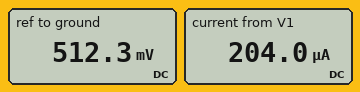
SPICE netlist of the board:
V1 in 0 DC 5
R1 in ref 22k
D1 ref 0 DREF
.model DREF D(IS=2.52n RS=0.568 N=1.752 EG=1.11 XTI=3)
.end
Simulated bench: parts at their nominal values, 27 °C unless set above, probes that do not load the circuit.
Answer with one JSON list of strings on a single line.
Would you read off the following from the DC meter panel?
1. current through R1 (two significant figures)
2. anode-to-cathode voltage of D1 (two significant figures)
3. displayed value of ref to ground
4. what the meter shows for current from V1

["200 µA", "510 mV", "512.3 mV", "204.0 µA"]
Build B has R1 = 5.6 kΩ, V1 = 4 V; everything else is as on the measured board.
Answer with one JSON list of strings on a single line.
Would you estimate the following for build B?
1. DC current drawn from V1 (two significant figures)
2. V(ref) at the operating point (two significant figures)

["610 µA", "560 mV"]
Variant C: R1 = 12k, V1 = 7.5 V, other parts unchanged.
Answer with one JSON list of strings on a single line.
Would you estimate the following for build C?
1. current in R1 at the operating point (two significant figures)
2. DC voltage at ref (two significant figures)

["580 µA", "560 mV"]
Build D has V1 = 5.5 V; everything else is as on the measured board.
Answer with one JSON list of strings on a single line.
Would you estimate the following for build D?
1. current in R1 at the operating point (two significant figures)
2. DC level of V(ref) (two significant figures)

["230 µA", "520 mV"]
